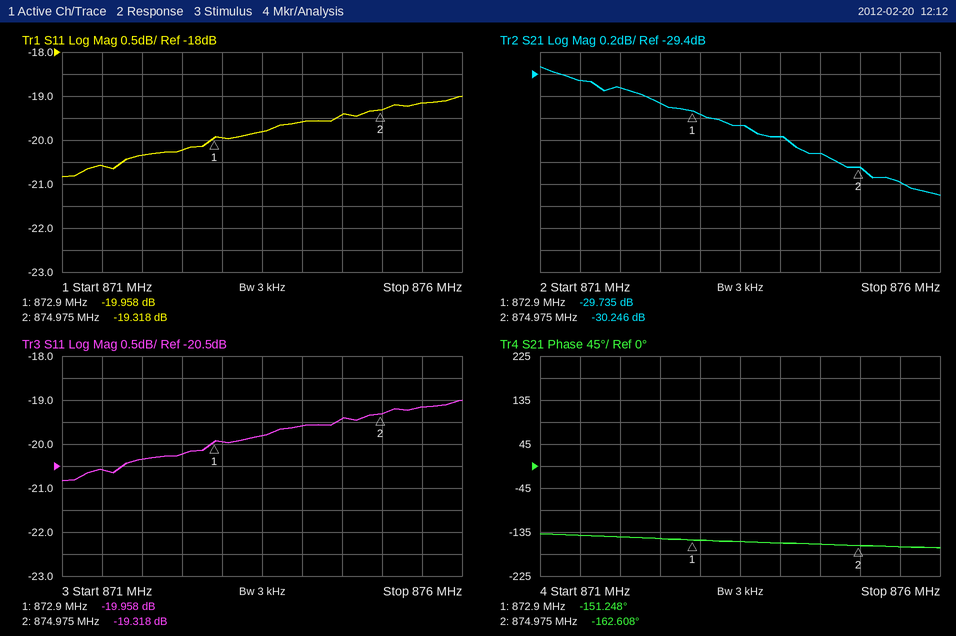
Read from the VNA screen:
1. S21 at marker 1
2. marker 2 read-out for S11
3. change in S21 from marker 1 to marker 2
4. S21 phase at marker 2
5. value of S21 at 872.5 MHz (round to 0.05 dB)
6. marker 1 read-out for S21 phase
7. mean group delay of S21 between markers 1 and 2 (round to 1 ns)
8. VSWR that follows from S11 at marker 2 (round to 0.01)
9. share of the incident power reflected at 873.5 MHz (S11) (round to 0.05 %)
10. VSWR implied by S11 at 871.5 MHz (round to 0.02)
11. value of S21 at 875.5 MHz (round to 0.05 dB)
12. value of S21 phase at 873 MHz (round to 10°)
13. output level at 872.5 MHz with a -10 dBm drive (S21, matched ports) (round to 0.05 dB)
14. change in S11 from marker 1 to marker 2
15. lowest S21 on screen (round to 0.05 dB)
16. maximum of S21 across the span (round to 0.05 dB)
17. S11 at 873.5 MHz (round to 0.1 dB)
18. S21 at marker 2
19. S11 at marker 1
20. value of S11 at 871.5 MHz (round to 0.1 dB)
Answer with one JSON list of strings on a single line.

["-29.735 dB", "-19.318 dB", "-0.511 dB", "-162.608°", "-29.65 dB", "-151.248°", "15 ns", "1.24", "1.05 %", "1.20", "-30.40 dB", "-150°", "-39.65 dBm", "0.640 dB", "-30.50 dB", "-29.35 dB", "-19.8 dB", "-30.246 dB", "-19.958 dB", "-20.6 dB"]
